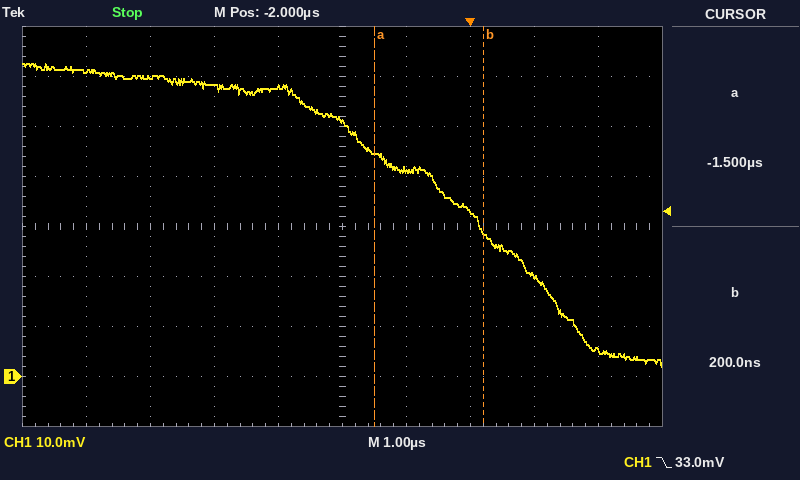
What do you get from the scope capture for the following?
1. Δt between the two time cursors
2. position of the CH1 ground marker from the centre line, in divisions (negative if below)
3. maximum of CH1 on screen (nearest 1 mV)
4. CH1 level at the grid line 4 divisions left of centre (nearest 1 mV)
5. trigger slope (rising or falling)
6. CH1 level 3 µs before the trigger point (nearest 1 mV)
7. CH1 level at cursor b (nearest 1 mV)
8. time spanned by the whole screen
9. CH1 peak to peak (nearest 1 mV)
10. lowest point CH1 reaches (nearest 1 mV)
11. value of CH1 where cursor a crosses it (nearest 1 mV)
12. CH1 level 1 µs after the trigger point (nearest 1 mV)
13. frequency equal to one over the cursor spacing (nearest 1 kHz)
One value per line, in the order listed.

1.7 µs
-3.0 div
63 mV
61 mV
falling
58 mV
29 mV
10 µs
61 mV
2 mV
45 mV
20 mV
588 kHz
